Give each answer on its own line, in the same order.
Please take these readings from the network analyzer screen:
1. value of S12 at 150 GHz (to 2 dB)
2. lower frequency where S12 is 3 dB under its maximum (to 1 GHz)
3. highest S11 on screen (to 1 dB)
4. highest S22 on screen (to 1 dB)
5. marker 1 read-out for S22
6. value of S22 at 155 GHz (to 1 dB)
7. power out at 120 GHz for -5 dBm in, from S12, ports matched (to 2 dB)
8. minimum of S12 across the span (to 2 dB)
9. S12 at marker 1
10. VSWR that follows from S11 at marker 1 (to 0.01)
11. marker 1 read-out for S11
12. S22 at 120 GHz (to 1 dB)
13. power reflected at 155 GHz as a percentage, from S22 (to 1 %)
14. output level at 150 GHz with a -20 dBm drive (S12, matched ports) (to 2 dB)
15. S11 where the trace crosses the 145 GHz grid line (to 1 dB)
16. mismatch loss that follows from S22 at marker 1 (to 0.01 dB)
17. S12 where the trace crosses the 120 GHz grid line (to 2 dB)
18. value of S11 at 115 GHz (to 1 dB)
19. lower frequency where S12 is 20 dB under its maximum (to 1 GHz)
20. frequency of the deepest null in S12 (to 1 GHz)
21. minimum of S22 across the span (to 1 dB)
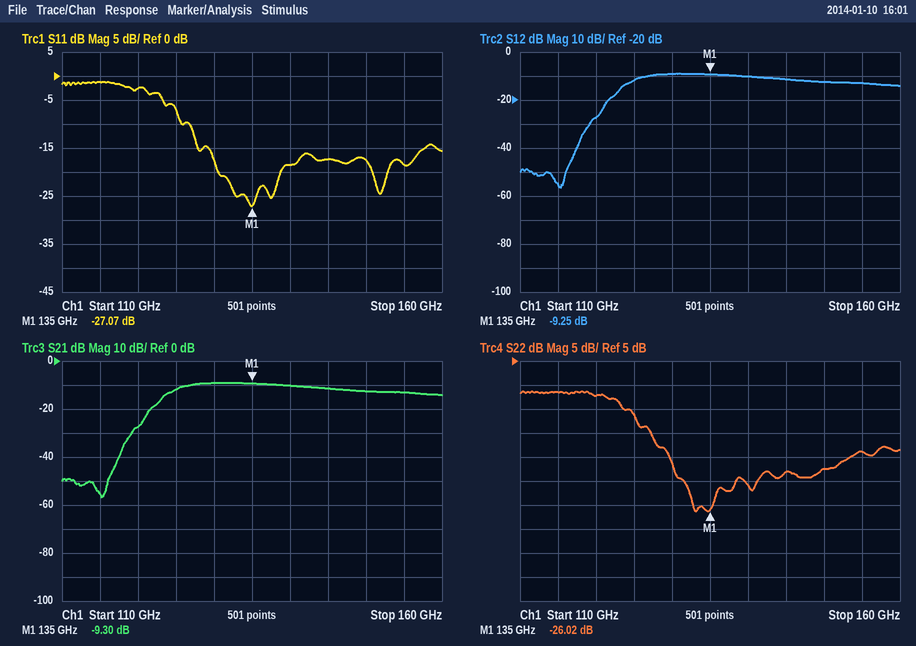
-12 dB
125 GHz
-1 dB
-1 dB
-26.02 dB
-14 dB
-32 dBm
-56 dB
-9.25 dB
1.09
-27.07 dB
-2 dB
4 %
-32 dBm
-17 dB
0.01 dB
-28 dB
-1 dB
119 GHz
115 GHz
-26 dB
